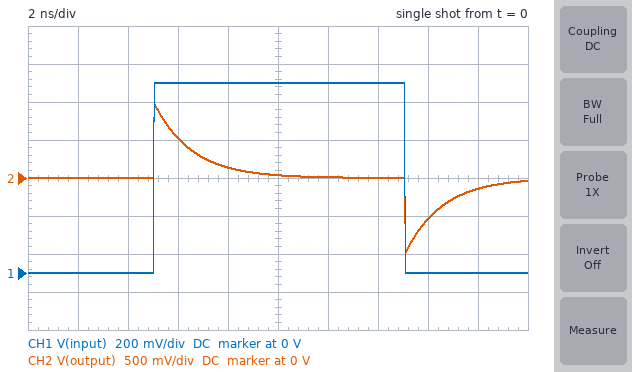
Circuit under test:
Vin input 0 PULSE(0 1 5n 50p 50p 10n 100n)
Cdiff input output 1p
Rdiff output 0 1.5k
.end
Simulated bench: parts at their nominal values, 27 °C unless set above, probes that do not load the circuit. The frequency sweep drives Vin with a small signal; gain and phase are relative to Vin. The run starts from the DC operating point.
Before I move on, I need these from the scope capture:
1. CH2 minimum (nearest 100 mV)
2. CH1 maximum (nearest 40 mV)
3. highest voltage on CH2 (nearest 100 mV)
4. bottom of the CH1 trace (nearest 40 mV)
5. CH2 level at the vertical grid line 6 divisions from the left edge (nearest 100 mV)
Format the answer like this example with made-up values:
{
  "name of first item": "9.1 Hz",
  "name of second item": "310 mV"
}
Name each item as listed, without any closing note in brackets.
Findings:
{
  "CH2 minimum": "-1.0 V",
  "CH1 maximum": "1.00 V",
  "highest voltage on CH2": "1.0 V",
  "bottom of the CH1 trace": "0 V",
  "CH2 level at the vertical grid line 6 divisions from the left edge": "0 V"
}
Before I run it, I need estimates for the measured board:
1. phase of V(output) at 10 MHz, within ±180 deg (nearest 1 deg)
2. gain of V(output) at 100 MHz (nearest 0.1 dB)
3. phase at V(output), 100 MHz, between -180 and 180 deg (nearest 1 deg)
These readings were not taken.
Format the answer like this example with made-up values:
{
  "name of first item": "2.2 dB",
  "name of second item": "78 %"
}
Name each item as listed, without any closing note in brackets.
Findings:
{
  "phase of V(output) at 10 MHz, within ±180 deg": "85 deg",
  "gain of V(output) at 100 MHz": "-3.3 dB",
  "phase at V(output), 100 MHz, between -180 and 180 deg": "47 deg"
}
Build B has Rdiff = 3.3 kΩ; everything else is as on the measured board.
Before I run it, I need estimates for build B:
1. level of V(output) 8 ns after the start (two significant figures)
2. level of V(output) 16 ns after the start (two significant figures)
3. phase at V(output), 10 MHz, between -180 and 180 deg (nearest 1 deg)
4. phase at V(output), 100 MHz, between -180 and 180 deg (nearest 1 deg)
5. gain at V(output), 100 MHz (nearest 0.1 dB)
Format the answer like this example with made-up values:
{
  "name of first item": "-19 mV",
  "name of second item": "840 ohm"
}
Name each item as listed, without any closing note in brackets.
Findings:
{
  "level of V(output) 8 ns after the start": "410 mV",
  "level of V(output) 16 ns after the start": "-720 mV",
  "phase at V(output), 10 MHz, between -180 and 180 deg": "78 deg",
  "phase at V(output), 100 MHz, between -180 and 180 deg": "26 deg",
  "gain at V(output), 100 MHz": "-0.9 dB"
}
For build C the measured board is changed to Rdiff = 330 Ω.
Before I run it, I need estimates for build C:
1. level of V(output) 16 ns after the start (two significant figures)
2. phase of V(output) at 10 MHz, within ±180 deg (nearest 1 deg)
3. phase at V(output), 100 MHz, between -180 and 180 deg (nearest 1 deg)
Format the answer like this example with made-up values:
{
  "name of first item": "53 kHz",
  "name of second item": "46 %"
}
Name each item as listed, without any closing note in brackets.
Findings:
{
  "level of V(output) 16 ns after the start": "-61 mV",
  "phase of V(output) at 10 MHz, within ±180 deg": "89 deg",
  "phase at V(output), 100 MHz, between -180 and 180 deg": "78 deg"
}
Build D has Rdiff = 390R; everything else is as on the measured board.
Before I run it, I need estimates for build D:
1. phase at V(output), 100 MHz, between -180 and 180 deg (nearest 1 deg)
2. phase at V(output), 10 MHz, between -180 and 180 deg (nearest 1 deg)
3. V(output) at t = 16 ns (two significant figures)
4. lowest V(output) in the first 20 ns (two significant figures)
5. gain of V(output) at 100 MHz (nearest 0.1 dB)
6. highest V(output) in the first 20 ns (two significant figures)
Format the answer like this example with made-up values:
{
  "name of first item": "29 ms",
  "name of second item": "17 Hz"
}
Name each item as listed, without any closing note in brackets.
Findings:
{
  "phase at V(output), 100 MHz, between -180 and 180 deg": "76 deg",
  "phase at V(output), 10 MHz, between -180 and 180 deg": "89 deg",
  "V(output) at t = 16 ns": "-93 mV",
  "lowest V(output) in the first 20 ns": "-940 mV",
  "gain of V(output) at 100 MHz": "-12.5 dB",
  "highest V(output) in the first 20 ns": "940 mV"
}
